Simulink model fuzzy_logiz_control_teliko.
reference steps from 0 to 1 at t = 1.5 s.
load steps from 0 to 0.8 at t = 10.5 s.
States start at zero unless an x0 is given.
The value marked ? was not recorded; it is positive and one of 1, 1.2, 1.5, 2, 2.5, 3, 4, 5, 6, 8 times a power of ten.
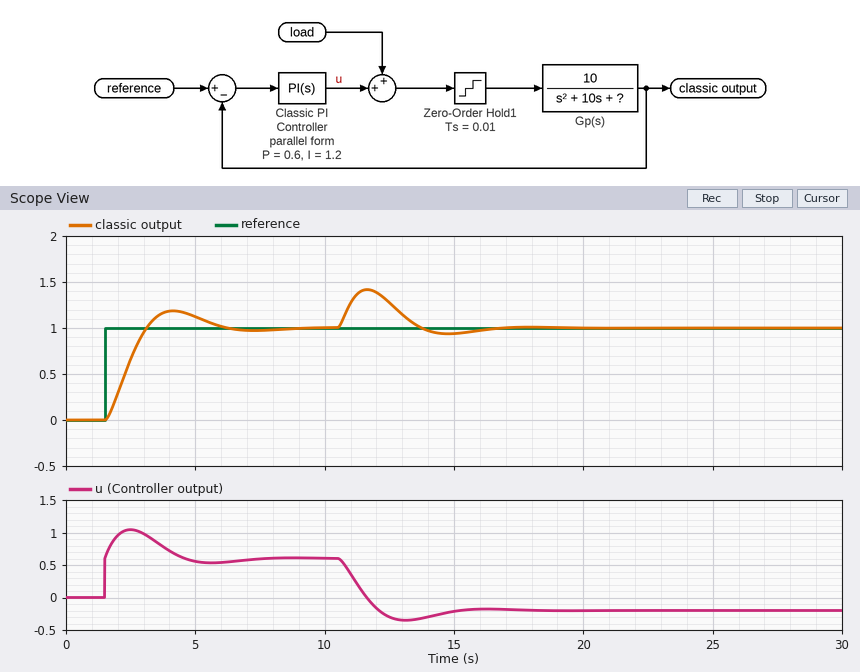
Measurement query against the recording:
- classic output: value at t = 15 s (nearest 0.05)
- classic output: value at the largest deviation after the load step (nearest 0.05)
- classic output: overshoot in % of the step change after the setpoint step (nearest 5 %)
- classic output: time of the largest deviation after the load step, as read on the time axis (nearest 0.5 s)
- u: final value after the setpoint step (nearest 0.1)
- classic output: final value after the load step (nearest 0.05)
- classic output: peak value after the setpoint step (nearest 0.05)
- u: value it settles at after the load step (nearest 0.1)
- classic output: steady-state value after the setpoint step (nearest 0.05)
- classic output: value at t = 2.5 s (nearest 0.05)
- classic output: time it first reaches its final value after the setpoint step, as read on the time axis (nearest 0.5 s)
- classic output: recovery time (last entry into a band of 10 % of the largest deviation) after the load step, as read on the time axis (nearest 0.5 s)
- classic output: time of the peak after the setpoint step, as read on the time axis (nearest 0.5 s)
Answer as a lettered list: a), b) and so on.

a) 0.95
b) 1.40
c) 20 %
d) 11.5 s
e) 0.6
f) 1.00
g) 1.20
h) -0.2
i) 1.00
j) 0.65
k) 3.0 s
l) 15.5 s
m) 4.0 s
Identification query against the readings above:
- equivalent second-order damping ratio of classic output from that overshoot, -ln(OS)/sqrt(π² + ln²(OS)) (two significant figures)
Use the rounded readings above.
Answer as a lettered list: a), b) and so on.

a) 0.46
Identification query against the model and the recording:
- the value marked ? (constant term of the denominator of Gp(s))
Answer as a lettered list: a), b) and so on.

a) 6
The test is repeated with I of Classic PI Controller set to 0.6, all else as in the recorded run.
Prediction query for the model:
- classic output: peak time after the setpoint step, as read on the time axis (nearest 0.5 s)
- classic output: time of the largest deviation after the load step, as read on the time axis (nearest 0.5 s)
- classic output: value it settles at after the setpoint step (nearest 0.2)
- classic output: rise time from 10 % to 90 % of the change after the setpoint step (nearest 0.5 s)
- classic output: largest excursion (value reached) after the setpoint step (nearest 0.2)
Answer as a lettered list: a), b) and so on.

a) 6.0 s
b) 12.0 s
c) 1.0
d) 2.0 s
e) 1.0
